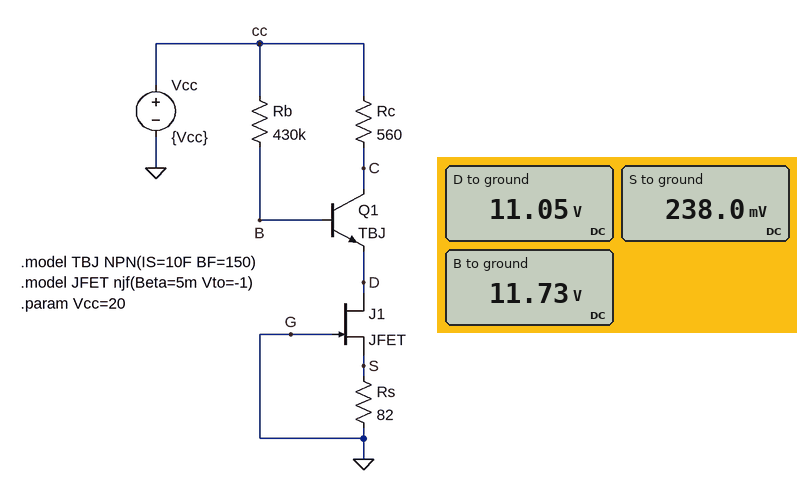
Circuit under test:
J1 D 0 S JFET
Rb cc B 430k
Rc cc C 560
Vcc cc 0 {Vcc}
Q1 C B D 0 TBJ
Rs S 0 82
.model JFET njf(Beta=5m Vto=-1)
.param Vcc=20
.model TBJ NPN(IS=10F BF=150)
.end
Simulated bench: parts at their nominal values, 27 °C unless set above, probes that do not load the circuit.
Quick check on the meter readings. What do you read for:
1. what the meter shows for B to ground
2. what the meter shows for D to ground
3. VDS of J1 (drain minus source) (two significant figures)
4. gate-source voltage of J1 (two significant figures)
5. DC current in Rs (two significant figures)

11.73 V
11.05 V
11 V
-240 mV
2.9 mA
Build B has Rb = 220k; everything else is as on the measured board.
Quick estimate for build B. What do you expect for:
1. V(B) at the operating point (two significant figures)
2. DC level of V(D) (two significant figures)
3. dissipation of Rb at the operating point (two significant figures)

16 V
15 V
81 µW
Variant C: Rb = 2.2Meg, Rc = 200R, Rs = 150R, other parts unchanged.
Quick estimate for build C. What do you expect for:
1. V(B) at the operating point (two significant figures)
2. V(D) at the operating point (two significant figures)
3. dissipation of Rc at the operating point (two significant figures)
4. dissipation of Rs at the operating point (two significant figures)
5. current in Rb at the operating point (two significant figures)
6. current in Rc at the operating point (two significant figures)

1.0 V
380 mV
330 µW
250 µW
8.6 µA
1.3 mA
